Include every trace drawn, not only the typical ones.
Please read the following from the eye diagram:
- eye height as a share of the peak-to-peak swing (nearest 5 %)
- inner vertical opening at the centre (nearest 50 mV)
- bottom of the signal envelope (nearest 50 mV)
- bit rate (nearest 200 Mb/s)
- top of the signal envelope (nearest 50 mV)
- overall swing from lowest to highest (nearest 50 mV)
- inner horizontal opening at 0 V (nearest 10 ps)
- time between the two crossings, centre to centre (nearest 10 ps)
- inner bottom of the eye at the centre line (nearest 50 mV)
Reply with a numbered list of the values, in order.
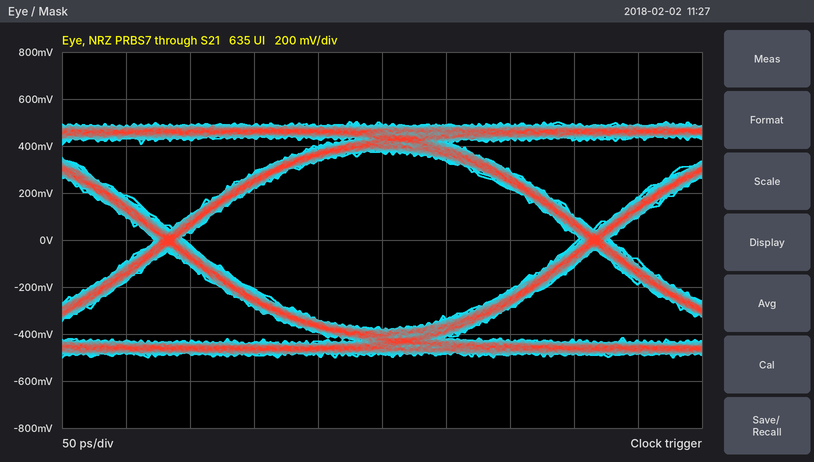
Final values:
1. 75 %
2. 750 mV
3. -500 mV
4. 3.0 Gb/s
5. 500 mV
6. 1.00 V
7. 310 ps
8. 330 ps
9. -400 mV
